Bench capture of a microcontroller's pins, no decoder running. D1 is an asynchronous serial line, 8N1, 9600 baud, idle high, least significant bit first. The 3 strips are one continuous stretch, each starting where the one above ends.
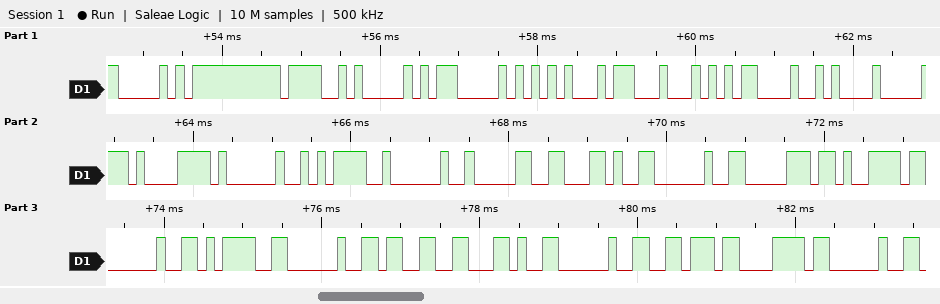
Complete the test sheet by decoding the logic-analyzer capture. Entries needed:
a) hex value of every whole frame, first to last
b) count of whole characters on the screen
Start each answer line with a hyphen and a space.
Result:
- 50 4F 50 50 45 44 0D 0A 70 78 20 3D 20 30 2C 20 70 79 20 3D 20 33 2C 20 76 78 20
- 27
